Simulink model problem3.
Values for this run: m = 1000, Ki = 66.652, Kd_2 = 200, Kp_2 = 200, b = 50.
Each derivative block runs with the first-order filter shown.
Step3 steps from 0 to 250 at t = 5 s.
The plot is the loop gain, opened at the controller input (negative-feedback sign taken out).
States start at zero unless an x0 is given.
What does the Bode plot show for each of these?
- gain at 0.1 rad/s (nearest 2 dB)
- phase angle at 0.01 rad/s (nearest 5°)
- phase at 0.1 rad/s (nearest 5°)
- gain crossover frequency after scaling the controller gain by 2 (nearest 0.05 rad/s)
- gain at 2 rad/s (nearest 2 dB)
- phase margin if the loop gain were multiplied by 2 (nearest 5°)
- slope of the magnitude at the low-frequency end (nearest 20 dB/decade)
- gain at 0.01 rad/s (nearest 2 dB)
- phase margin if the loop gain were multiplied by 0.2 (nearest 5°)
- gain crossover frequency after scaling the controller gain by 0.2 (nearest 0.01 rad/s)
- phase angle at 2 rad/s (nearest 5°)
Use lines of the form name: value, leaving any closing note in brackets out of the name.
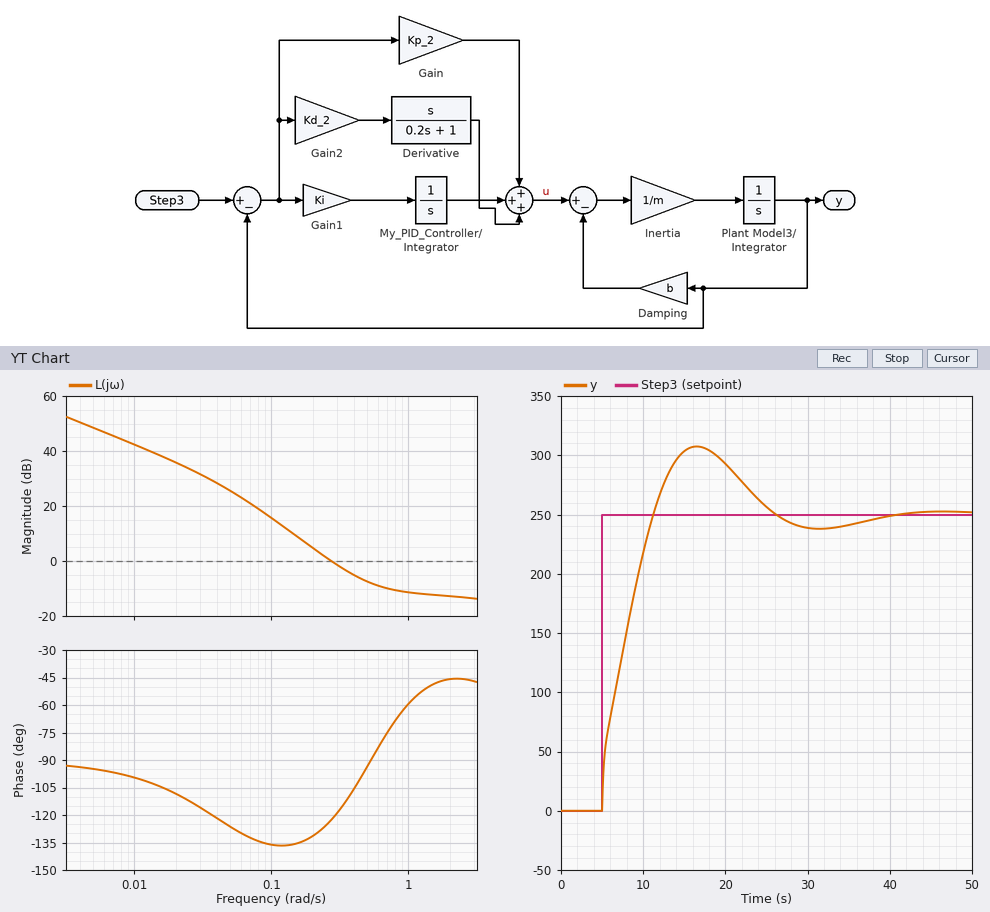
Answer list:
gain at 0.1 rad/s: 16 dB
phase angle at 0.01 rad/s: -100°
phase at 0.1 rad/s: -135°
gain crossover frequency after scaling the controller gain by 2: 0.45 rad/s
gain at 2 rad/s: -12 dB
phase margin if the loop gain were multiplied by 2: 80°
slope of the magnitude at the low-frequency end: -20 dB/decade
gain at 0.01 rad/s: 42 dB
phase margin if the loop gain were multiplied by 0.2: 45°
gain crossover frequency after scaling the controller gain by 0.2: 0.11 rad/s
phase angle at 2 rad/s: -45°
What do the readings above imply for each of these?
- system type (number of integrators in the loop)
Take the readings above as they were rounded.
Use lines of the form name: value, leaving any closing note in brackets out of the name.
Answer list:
system type: 1
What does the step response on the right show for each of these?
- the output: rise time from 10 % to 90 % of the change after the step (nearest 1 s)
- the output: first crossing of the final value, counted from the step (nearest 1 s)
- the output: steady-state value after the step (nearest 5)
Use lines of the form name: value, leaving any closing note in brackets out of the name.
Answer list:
the output: rise time from 10 % to 90 % of the change after the step: 5 s
the output: first crossing of the final value, counted from the step: 6 s
the output: steady-state value after the step: 250
